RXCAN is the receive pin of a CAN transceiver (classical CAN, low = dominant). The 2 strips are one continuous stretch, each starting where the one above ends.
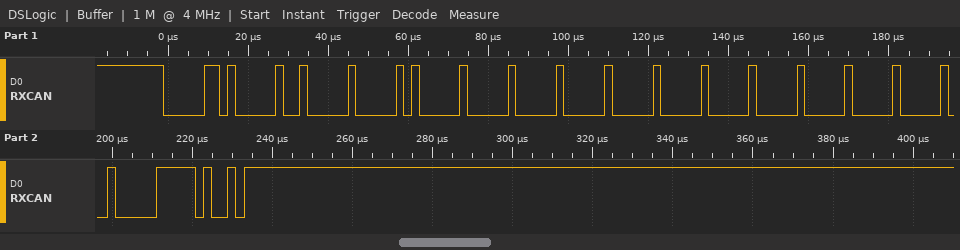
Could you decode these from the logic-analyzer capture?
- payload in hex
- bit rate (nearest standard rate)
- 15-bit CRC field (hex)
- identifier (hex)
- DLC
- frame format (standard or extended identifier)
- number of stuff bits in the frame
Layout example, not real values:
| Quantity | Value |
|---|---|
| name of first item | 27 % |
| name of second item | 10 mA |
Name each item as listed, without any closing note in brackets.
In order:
| Quantity | Value |
|---|---|
| payload in hex | 00 80 00 00 00 00 00 00 |
| bit rate | 500 kbit/s |
| 15-bit CRC field | 0x107C |
| identifier | 0x050 |
| DLC | 8 |
| frame format | standard |
| number of stuff bits in the frame | 17 |
